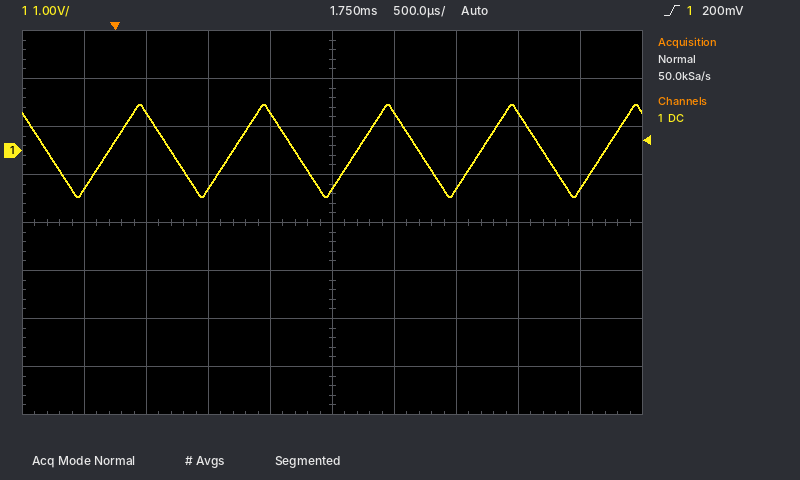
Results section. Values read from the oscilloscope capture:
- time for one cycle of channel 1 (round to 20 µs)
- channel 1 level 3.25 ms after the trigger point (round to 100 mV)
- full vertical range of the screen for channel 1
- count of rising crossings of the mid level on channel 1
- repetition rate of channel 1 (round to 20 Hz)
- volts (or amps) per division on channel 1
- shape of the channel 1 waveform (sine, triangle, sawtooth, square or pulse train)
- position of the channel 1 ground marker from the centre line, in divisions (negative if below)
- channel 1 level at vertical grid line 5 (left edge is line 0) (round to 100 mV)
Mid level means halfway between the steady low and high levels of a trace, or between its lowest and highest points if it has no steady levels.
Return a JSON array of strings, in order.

["1.00 ms", "800 mV", "8 V", "5", "1.00 kHz", "1 V", "triangle", "+1.5 div", "-800 mV"]
